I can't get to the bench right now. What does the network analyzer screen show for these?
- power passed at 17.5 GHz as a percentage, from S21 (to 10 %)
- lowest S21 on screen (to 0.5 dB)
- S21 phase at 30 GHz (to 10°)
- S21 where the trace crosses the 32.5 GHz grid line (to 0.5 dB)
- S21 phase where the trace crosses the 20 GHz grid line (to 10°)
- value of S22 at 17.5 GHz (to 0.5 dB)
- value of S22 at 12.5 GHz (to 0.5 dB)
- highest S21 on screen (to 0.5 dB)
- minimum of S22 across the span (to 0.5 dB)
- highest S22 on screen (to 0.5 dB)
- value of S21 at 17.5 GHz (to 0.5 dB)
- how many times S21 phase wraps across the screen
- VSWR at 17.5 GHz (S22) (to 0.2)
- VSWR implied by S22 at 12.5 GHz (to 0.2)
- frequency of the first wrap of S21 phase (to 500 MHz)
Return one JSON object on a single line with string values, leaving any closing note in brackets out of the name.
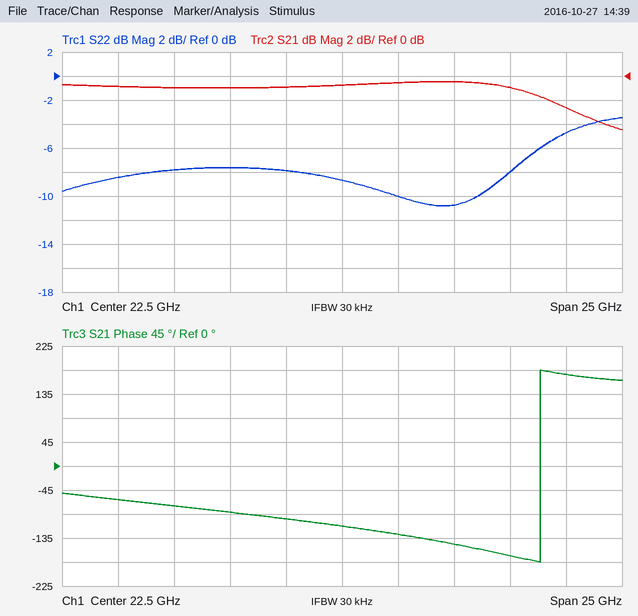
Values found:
{"power passed at 17.5 GHz as a percentage, from S21": "80 %", "lowest S21 on screen": "-4.5 dB", "S21 phase at 30 GHz": "-170°", "S21 where the trace crosses the 32.5 GHz grid line": "-2.5 dB", "S21 phase where the trace crosses the 20 GHz grid line": "-100°", "value of S22 at 17.5 GHz": "-7.5 dB", "value of S22 at 12.5 GHz": "-8.5 dB", "highest S21 on screen": "-0.5 dB", "minimum of S22 across the span": "-11.0 dB", "highest S22 on screen": "-3.5 dB", "value of S21 at 17.5 GHz": "-1.0 dB", "how many times S21 phase wraps across the screen": "1", "VSWR at 17.5 GHz (S22)": "2.4", "VSWR implied by S22 at 12.5 GHz": "2.2", "frequency of the first wrap of S21 phase": "31.5 GHz"}
